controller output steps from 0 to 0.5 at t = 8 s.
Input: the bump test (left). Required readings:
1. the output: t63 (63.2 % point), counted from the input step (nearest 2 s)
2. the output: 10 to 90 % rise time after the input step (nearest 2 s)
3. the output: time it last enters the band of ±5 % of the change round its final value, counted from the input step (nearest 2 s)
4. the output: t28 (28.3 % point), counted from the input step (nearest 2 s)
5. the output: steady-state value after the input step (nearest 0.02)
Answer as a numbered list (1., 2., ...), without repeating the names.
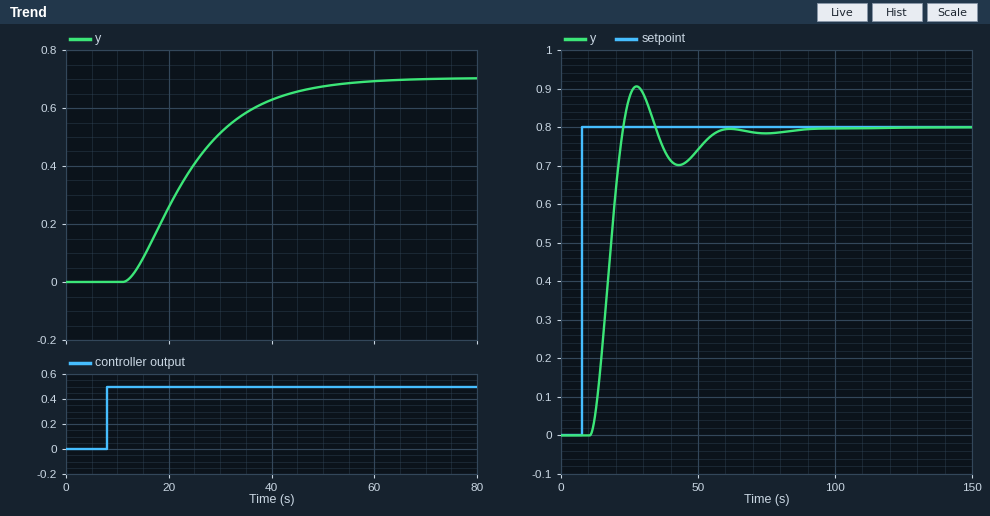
1. 18 s
2. 26 s
3. 40 s
4. 10 s
5. 0.70
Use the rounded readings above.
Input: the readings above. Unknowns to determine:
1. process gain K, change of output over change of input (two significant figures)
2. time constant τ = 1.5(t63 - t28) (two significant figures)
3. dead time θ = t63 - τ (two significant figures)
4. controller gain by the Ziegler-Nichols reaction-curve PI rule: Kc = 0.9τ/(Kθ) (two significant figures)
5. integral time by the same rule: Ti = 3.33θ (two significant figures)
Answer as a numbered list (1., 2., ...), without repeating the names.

1. 1.4
2. 12 s
3. 6.0 s
4. 1.3
5. 20 s
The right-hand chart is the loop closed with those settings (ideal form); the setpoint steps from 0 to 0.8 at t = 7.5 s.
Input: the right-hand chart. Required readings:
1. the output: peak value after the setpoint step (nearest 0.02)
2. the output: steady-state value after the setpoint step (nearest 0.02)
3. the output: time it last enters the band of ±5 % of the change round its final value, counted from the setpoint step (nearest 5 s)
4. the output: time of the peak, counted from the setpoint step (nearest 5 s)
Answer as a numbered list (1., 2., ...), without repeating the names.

1. 0.90
2. 0.80
3. 45 s
4. 20 s
